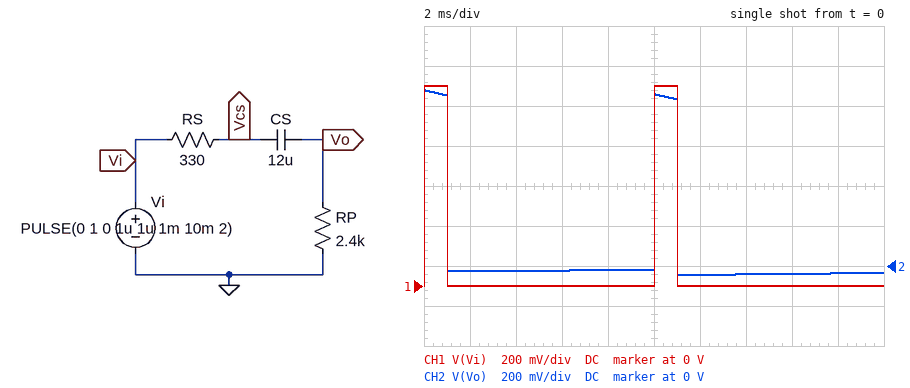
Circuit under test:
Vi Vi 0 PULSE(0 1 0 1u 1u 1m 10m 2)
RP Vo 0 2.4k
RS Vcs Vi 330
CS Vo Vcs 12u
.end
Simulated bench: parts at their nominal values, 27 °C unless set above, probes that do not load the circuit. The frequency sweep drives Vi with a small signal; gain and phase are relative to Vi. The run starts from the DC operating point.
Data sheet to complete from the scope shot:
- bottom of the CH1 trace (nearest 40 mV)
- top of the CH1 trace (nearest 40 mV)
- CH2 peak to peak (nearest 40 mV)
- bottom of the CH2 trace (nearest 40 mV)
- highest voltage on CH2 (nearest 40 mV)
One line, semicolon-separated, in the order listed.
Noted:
0 V; 1.00 V; 920 mV; -40 mV; 880 mV
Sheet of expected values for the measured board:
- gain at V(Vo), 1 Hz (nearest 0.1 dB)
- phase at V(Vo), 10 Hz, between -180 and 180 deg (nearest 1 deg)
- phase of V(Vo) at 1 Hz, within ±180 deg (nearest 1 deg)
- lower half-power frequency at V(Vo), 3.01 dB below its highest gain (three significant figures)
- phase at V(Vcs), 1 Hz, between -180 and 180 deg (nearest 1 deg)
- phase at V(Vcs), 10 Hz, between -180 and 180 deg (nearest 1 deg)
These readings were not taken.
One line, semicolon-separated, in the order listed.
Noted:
-15.0 dB; 26 deg; 78 deg; 4.86 Hz; -1 deg; -3 deg
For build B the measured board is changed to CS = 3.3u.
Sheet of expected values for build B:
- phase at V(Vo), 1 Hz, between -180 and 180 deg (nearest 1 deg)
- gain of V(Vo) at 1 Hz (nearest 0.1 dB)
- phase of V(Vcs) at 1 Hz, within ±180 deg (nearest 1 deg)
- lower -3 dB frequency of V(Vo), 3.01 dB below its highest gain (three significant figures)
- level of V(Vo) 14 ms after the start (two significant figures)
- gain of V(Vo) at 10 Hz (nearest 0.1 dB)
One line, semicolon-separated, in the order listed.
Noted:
87 deg; -26.1 dB; 0 deg; 17.7 Hz; -88 mV; -7.3 dB
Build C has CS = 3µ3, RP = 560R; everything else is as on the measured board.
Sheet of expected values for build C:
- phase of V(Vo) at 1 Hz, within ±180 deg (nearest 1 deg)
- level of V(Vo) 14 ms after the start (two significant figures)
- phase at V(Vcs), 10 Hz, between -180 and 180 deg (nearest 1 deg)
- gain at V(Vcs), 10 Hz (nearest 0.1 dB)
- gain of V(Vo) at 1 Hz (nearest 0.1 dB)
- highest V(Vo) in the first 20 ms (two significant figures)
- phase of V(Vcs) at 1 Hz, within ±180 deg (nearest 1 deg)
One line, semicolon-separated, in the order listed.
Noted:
89 deg; -68 mV; -4 deg; -0.1 dB; -38.7 dB; 630 mV; 0 deg
